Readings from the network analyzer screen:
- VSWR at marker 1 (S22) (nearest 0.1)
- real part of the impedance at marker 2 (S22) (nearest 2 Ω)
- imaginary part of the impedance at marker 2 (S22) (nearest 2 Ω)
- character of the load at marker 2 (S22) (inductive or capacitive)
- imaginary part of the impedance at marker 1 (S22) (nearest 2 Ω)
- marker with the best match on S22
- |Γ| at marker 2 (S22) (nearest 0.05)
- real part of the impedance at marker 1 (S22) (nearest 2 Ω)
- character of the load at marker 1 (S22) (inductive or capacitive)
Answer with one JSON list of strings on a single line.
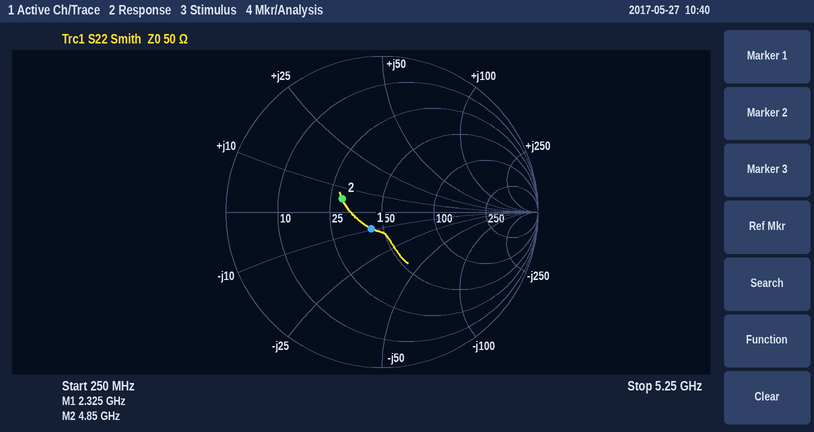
["1.3", "30 Ω", "+6 Ω", "inductive", "-10 Ω", "marker 1", "0.25", "42 Ω", "capacitive"]
